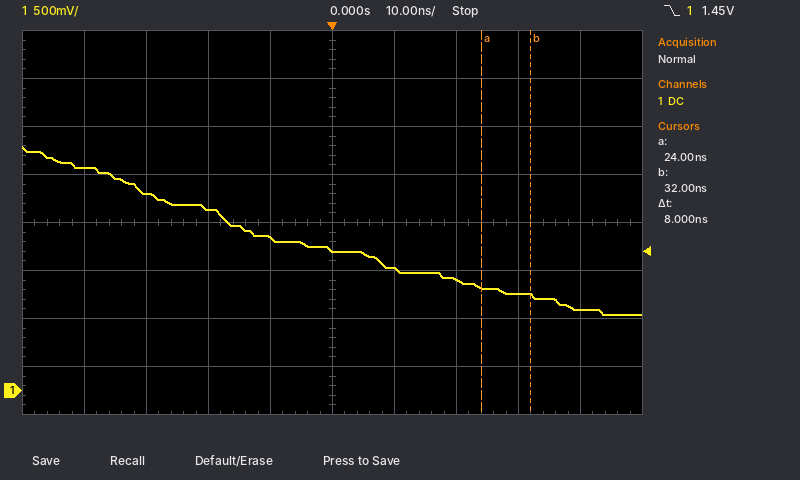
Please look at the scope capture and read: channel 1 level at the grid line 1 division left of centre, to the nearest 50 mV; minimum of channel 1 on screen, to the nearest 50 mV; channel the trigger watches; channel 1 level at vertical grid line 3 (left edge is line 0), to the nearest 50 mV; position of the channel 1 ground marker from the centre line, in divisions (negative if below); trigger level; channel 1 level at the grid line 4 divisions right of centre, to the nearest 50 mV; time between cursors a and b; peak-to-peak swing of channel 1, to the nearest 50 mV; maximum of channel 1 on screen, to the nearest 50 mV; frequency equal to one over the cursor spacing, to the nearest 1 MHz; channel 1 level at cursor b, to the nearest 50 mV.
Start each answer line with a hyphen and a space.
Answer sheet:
- 1.60 V
- 800 mV
- channel 1
- 1.90 V
- -3.5 div
- 1.45 V
- 850 mV
- 8 ns
- 1.75 V
- 2.55 V
- 125 MHz
- 1.00 V
